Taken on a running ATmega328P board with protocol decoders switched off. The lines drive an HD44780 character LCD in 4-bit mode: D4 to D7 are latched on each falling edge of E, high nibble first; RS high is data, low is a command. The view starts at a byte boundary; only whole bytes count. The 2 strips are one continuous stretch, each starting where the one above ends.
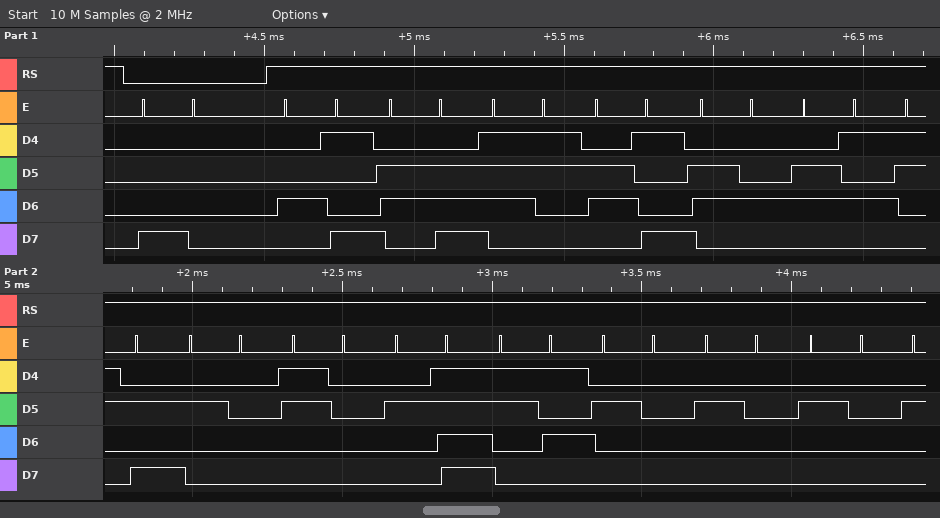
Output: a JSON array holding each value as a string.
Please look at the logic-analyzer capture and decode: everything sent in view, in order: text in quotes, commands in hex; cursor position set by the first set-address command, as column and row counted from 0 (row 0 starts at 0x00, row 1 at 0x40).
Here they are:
["0x80 \"Inside: 0/5   \"", "column 0, row 0"]
